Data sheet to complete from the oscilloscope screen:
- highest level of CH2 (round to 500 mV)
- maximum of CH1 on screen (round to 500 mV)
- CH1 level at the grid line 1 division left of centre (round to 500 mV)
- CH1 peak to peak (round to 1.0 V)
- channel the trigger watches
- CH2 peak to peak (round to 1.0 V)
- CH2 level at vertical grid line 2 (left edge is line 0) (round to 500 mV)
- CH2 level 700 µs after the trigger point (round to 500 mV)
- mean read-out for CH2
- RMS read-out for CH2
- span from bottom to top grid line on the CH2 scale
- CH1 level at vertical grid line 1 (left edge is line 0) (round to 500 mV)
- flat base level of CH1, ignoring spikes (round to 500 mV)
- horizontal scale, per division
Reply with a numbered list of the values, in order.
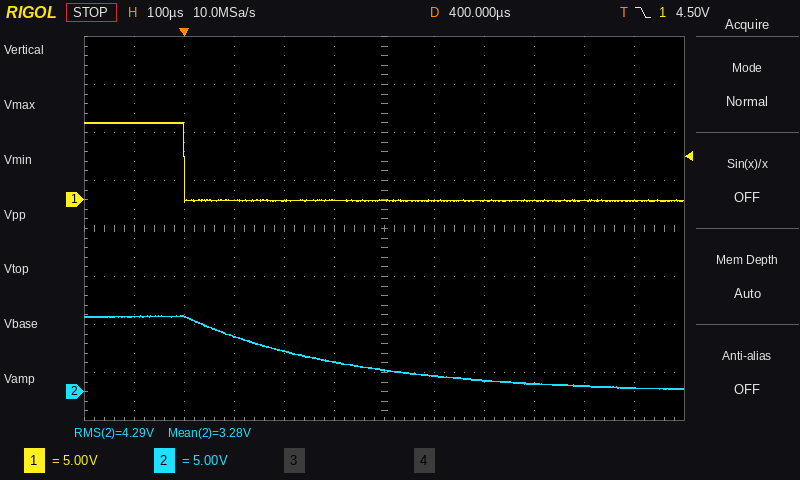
1. 8.0 V
2. 8.0 V
3. 0.0 V
4. 8.0 V
5. CH1
6. 8.0 V
7. 8.0 V
8. 1.0 V
9. 3.28 V
10. 4.29 V
11. 40 V
12. 8.0 V
13. 0.0 V
14. 100 µs
